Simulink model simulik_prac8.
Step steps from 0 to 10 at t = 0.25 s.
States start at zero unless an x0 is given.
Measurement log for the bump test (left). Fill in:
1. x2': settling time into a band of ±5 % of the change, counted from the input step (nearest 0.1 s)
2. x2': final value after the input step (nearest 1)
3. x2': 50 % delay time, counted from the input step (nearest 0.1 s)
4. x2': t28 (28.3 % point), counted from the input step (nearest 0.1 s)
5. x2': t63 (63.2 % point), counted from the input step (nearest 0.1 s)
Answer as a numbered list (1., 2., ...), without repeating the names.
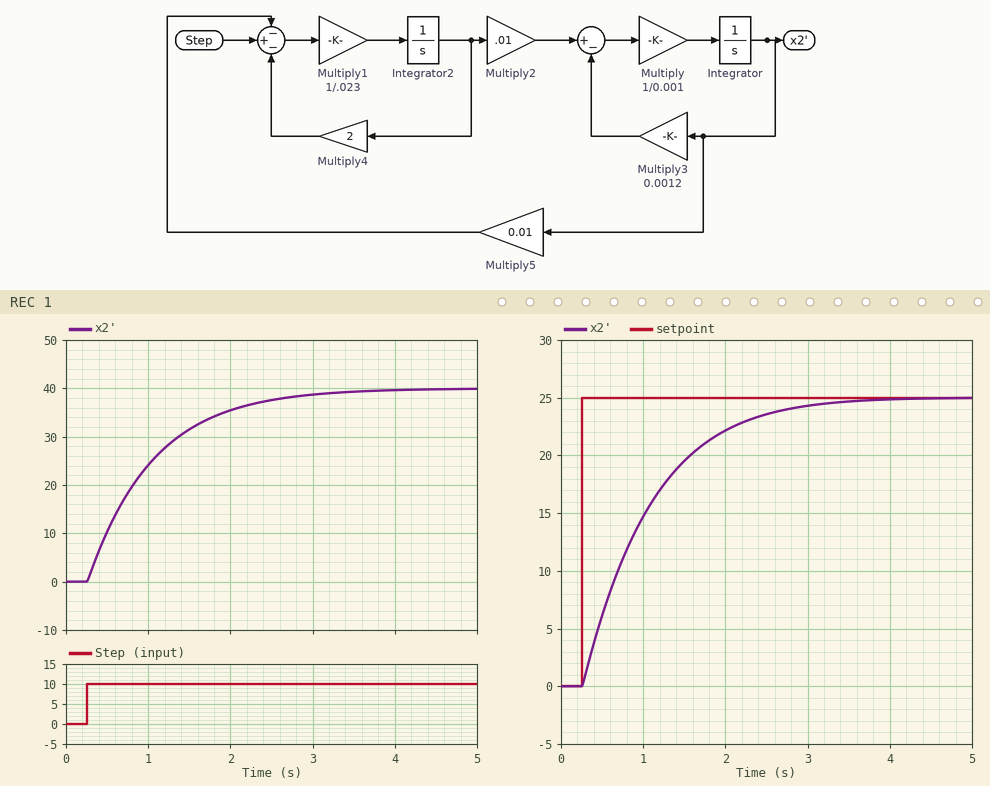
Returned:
1. 2.4 s
2. 40
3. 0.6 s
4. 0.3 s
5. 0.8 s
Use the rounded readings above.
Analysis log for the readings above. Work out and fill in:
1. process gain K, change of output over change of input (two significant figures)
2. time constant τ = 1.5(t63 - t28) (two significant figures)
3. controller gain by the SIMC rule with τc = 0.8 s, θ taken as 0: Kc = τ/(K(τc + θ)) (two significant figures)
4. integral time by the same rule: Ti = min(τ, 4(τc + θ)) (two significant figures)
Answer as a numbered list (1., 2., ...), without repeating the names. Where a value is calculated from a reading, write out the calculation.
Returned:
1. (40 - 0) / 10 = 4.0
2. 1.5 × (0.8 - 0.3) = 0.75 s
3. 0.75 / (4 × (0.8 + 0)) = 0.23
4. min(0.75, 4 × (0.8 + 0)) = 0.75 s
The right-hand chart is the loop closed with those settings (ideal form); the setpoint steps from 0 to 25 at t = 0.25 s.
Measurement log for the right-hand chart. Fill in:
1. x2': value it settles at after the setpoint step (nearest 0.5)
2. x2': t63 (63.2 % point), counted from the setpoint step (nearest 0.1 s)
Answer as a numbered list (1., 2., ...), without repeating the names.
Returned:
1. 25.0
2. 0.8 s
